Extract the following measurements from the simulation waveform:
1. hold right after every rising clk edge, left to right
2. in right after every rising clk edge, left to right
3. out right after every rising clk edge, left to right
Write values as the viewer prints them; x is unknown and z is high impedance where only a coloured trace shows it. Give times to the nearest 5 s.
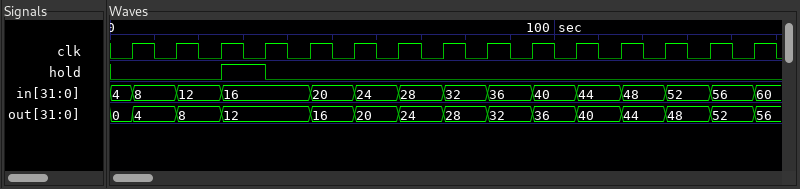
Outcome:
0 0 1 0 0 0 0 0 0 0 0 0 0 0 0
8, 12, 16, 16, 20, 24, 28, 32, 36, 40, 44, 48, 52, 56, 60
4, 8, 12, 12, 16, 20, 24, 28, 32, 36, 40, 44, 48, 52, 56
